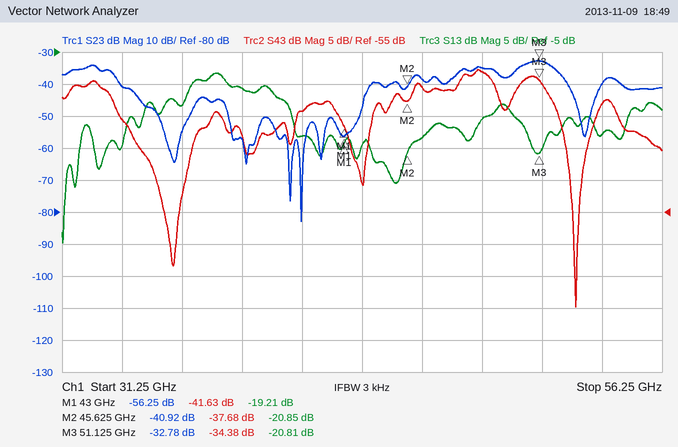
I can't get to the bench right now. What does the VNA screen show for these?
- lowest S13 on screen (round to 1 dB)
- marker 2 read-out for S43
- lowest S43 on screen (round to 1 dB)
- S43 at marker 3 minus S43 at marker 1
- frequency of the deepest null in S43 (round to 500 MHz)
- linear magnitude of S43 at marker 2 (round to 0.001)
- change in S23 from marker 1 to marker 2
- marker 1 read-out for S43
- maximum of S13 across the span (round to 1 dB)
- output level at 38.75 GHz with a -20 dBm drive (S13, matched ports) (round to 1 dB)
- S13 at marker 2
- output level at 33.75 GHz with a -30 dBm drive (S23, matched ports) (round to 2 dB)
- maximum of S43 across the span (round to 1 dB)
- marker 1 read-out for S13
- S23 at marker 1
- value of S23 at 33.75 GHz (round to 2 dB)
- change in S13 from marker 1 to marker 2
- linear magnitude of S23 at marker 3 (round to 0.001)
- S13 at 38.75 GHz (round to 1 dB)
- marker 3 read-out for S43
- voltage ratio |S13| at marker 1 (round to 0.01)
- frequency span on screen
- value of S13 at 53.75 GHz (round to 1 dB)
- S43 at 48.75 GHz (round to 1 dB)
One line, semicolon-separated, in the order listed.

-35 dB; -37.68 dB; -70 dB; 7.25 dB; 52.5 GHz; 0.013; 15.33 dB; -41.63 dB; -8 dB; -31 dBm; -20.85 dB; -70 dBm; -33 dB; -19.21 dB; -56.25 dB; -40 dB; -1.64 dB; 0.023; -11 dB; -34.38 dB; 0.11; 25 GHz; -18 dB; -33 dB
